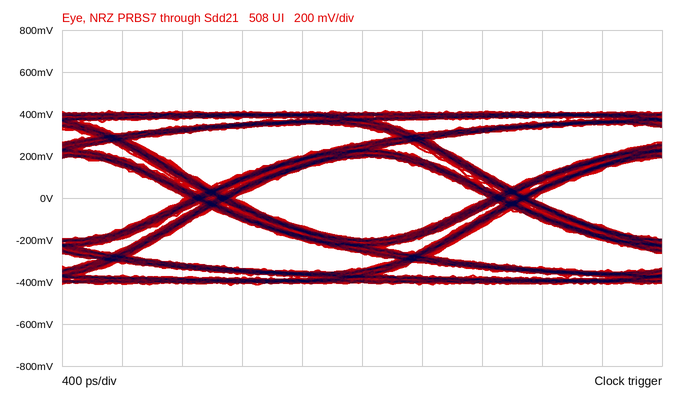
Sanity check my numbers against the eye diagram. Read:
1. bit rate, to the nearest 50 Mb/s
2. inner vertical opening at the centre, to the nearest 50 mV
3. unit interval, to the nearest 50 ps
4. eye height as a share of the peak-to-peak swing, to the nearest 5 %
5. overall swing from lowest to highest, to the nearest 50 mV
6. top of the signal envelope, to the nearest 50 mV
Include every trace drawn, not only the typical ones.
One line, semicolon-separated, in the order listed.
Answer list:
500 Mb/s; 400 mV; 2.00 ns; 45 %; 850 mV; 400 mV
